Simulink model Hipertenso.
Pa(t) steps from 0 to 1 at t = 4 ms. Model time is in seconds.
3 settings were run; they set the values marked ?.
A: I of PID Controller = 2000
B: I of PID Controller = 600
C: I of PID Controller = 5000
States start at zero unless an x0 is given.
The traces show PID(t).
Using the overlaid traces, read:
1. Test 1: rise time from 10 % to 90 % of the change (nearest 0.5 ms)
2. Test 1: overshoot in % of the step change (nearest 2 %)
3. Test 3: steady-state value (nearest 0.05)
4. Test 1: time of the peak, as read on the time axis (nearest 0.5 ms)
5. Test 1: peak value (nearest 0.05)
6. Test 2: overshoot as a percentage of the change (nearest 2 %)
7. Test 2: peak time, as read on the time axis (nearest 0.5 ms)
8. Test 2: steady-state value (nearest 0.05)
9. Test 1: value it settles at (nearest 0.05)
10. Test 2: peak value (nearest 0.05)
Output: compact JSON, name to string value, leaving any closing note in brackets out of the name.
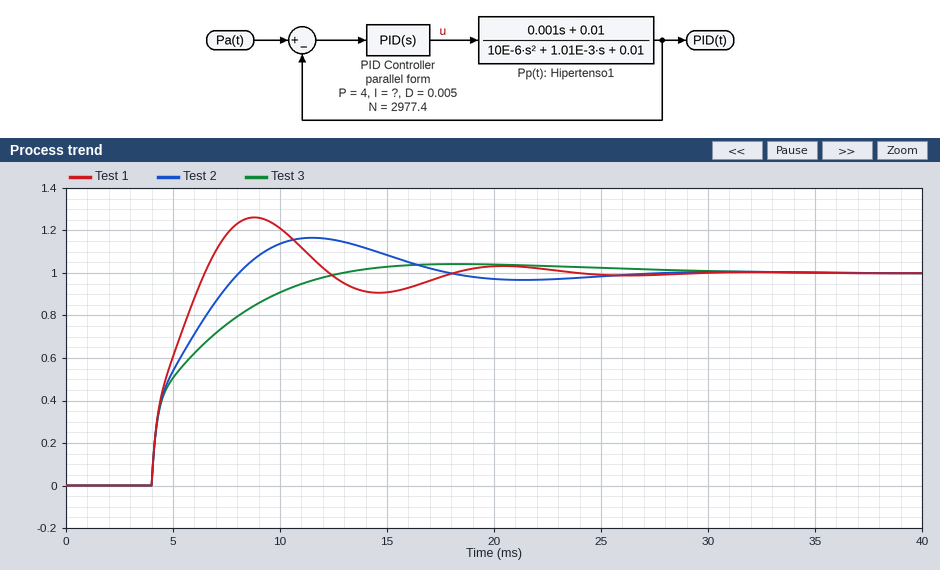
{"Test 1: rise time from 10 % to 90 % of the change": "2.0 ms", "Test 1: overshoot in % of the step change": "26 %", "Test 3: steady-state value": "1.00", "Test 1: time of the peak, as read on the time axis": "9.0 ms", "Test 1: peak value": "1.25", "Test 2: overshoot as a percentage of the change": "16 %", "Test 2: peak time, as read on the time axis": "11.5 ms", "Test 2: steady-state value": "1.00", "Test 1: value it settles at": "1.00", "Test 2: peak value": "1.15"}
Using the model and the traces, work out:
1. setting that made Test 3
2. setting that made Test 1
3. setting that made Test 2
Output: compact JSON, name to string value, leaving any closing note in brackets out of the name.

{"setting that made Test 3": "B", "setting that made Test 1": "C", "setting that made Test 2": "A"}
